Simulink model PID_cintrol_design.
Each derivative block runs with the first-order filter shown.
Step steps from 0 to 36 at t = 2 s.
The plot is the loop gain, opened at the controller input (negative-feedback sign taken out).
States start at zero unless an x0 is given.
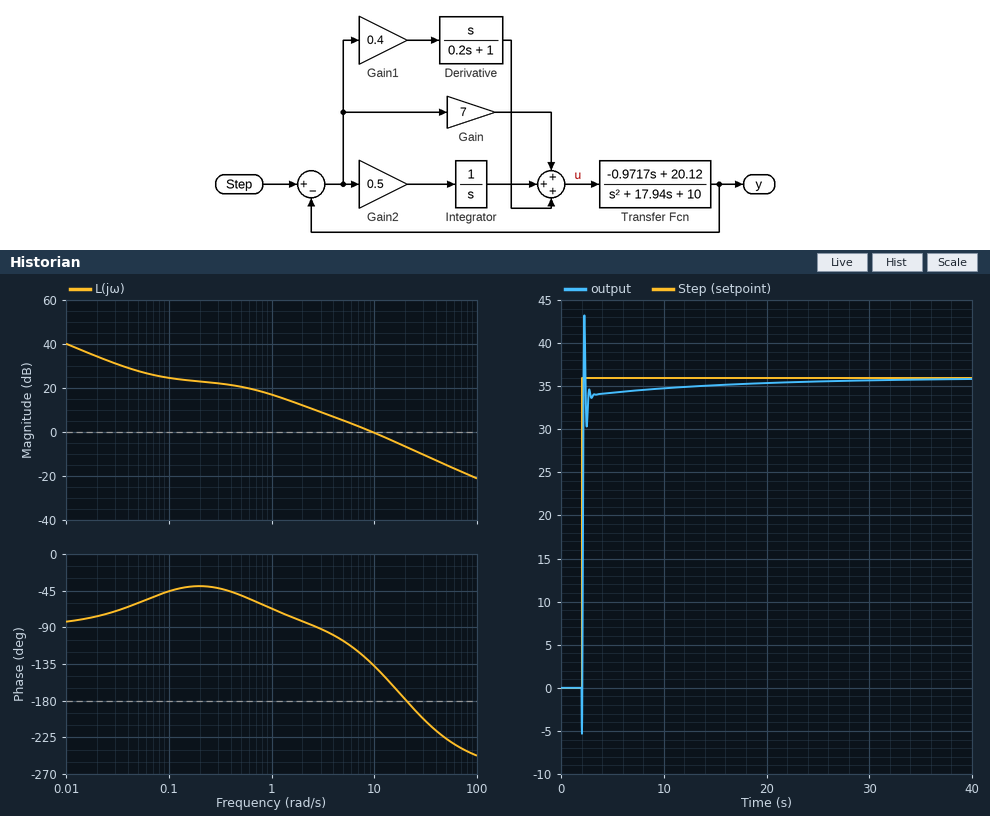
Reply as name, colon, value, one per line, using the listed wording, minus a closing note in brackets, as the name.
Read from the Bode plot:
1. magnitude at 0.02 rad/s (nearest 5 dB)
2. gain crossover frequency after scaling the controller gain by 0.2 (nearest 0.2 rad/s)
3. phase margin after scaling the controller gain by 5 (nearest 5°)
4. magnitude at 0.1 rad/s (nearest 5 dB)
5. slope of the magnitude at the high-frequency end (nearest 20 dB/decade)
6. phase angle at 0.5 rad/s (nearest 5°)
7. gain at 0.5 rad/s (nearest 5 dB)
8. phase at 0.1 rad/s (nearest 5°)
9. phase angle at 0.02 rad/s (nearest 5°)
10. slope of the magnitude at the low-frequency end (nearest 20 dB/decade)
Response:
magnitude at 0.02 rad/s: 35 dB
gain crossover frequency after scaling the controller gain by 0.2: 1.6 rad/s
phase margin after scaling the controller gain by 5: -40°
magnitude at 0.1 rad/s: 25 dB
slope of the magnitude at the high-frequency end: -20 dB/decade
phase angle at 0.5 rad/s: -50°
gain at 0.5 rad/s: 20 dB
phase at 0.1 rad/s: -45°
phase angle at 0.02 rad/s: -75°
slope of the magnitude at the low-frequency end: -20 dB/decade
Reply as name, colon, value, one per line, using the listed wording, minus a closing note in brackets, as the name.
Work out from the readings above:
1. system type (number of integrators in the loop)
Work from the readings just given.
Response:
system type: 1
